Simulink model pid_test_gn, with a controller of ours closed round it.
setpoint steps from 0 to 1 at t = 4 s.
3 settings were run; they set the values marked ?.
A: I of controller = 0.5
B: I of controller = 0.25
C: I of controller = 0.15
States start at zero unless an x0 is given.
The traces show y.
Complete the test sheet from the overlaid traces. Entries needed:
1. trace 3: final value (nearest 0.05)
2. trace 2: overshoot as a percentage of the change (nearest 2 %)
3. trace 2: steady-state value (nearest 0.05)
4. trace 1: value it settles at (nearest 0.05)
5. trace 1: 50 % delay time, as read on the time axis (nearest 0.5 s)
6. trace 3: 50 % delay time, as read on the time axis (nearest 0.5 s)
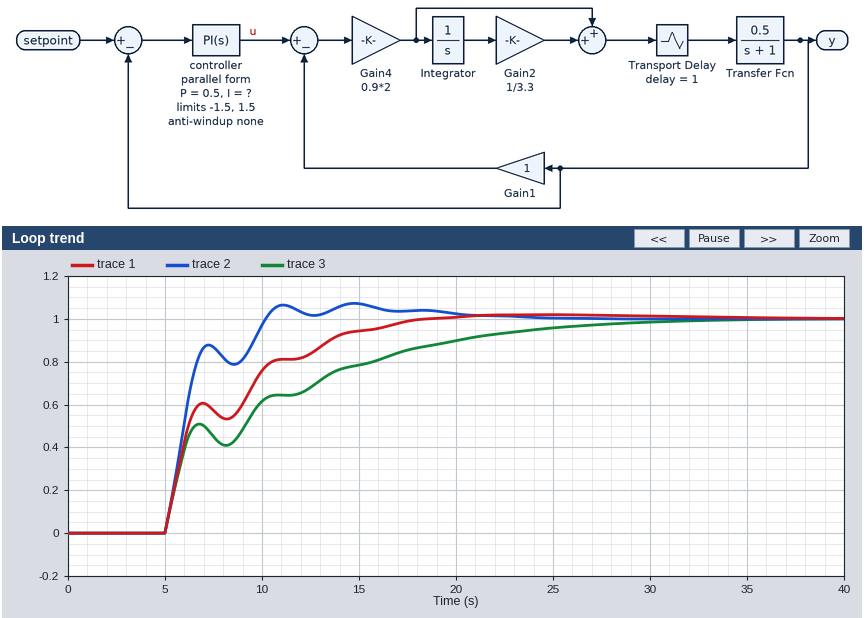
1.00
8 %
1.00
1.00
6.0 s
6.5 s
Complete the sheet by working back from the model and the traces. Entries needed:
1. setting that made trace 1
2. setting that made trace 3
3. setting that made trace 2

B
C
A
